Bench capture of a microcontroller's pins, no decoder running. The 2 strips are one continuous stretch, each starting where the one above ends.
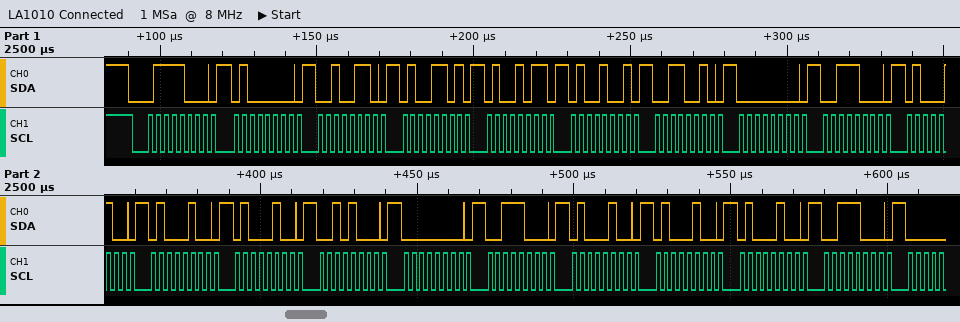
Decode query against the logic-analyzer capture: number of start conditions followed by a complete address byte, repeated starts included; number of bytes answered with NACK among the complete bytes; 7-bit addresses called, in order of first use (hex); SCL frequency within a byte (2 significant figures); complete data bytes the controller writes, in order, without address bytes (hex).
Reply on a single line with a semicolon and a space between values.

1; 0; 0x3C; 400 kHz; 40 26 4D 4B 49 32 00 38 44 44 44 28 00 38 44 44 44 38
